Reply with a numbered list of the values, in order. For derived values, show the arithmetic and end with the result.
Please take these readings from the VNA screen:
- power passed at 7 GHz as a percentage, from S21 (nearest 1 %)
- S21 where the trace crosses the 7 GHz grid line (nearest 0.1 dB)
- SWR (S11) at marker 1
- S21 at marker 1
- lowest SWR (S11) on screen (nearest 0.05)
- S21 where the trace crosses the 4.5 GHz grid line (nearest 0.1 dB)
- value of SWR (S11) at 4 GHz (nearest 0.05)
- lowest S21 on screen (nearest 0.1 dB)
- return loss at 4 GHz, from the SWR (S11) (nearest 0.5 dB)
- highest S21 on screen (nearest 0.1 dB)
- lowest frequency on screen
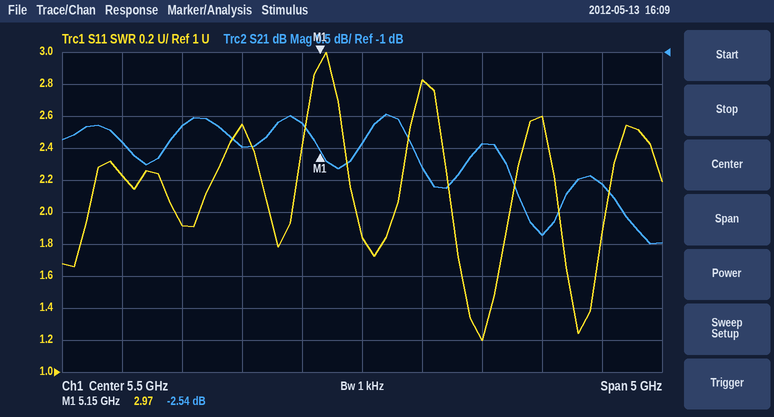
1. 10^(-3.9/10) ≈ 41 %
2. -3.9 dB
3. 2.97
4. -2.54 dB
5. 1.20
6. -2.5 dB
7. 1.90
8. -4.0 dB
9. −20 log10((1.9 − 1)/(1.9 + 1)) ≈ 10.2 dB, so 10.0 dB to the nearest 0.5 dB
10. -2.0 dB
11. 3 GHz
